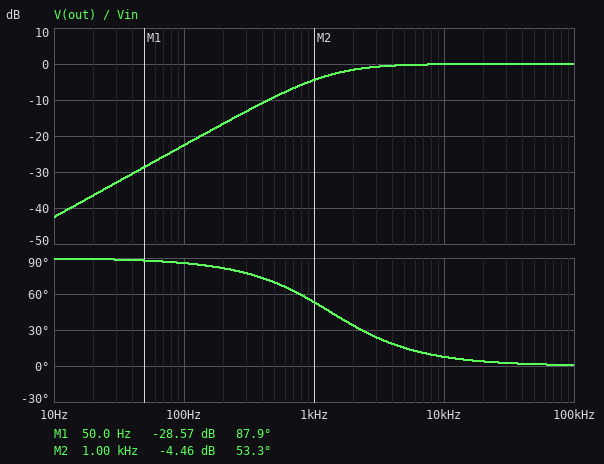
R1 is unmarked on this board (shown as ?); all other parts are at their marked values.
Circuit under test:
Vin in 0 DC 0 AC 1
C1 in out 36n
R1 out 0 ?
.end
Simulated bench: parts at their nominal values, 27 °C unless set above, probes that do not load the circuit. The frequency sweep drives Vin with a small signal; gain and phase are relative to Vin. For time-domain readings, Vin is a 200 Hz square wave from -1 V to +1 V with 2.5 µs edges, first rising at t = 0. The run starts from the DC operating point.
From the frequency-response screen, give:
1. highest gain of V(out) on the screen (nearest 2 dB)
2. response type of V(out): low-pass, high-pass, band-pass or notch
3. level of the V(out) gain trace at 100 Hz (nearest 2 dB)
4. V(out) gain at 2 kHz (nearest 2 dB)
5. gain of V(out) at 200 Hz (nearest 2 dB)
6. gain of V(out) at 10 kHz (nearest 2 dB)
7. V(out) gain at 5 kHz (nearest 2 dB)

0 dB
high-pass
-22 dB
-2 dB
-16 dB
0 dB
0 dB
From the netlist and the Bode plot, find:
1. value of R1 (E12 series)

3.3 kΩ
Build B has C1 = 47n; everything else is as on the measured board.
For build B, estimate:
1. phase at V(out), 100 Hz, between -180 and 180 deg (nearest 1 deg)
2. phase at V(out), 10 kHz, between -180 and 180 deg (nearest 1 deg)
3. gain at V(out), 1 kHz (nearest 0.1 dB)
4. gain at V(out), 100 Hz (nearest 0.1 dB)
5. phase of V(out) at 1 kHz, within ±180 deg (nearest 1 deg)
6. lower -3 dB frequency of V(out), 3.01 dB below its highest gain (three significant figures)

84 deg
6 deg
-3.1 dB
-20.3 dB
46 deg
1.03 kHz
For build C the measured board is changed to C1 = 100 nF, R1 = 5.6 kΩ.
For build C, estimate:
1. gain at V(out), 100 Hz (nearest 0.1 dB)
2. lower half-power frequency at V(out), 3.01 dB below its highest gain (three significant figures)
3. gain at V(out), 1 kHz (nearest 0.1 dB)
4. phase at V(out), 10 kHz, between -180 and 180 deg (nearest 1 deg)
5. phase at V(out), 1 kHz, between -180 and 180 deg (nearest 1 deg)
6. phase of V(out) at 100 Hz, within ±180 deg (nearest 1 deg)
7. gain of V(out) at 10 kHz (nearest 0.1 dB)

-9.6 dB
284 Hz
-0.3 dB
2 deg
16 deg
71 deg
0 dB
